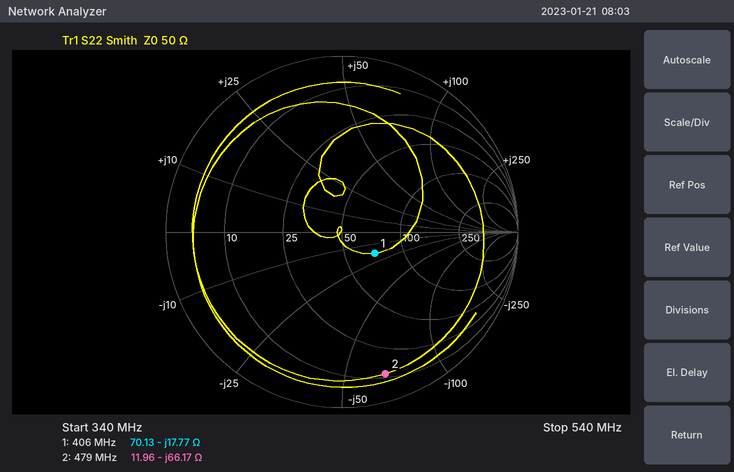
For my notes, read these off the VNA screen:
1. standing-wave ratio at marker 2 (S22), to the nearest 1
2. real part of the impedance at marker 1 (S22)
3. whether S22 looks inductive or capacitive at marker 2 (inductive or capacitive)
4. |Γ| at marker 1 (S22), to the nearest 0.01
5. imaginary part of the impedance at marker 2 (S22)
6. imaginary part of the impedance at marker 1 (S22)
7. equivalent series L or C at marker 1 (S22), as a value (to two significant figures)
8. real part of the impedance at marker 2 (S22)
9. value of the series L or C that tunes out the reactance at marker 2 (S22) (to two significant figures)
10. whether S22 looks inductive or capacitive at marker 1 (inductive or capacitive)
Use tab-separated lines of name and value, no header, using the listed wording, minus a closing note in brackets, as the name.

standing-wave ratio at marker 2 (S22), to the nearest 1	12
real part of the impedance at marker 1	70.13 Ω
whether S22 looks inductive or capacitive at marker 2	capacitive
|Γ| at marker 1 (S22), to the nearest 0.01	0.22
imaginary part of the impedance at marker 2	-66.17 Ω
imaginary part of the impedance at marker 1	-17.77 Ω
equivalent series L or C at marker 1 (S22), as a value	22 pF
real part of the impedance at marker 2	11.96 Ω
value of the series L or C that tunes out the reactance at marker 2 (S22)	22 nH
whether S22 looks inductive or capacitive at marker 1	capacitive
